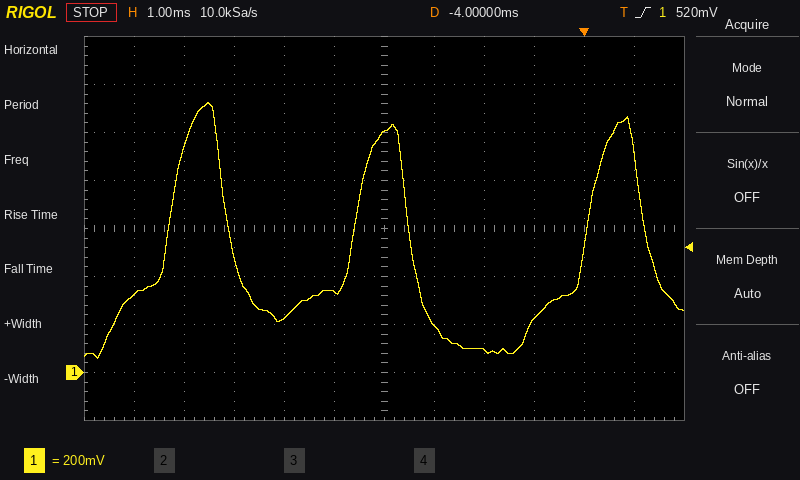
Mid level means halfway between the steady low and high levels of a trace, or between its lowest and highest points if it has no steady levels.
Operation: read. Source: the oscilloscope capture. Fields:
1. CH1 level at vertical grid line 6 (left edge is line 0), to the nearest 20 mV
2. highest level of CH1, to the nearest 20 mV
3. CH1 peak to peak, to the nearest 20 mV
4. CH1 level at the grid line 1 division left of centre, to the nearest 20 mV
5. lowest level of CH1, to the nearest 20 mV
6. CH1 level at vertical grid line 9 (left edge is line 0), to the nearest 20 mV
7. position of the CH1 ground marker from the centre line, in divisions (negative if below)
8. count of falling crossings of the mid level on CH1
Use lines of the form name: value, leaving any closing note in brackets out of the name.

CH1 level at vertical grid line 6 (left edge is line 0), to the nearest 20 mV: 1.00 V
highest level of CH1, to the nearest 20 mV: 1.12 V
CH1 peak to peak, to the nearest 20 mV: 1.06 V
CH1 level at the grid line 1 division left of centre, to the nearest 20 mV: 340 mV
lowest level of CH1, to the nearest 20 mV: 60 mV
CH1 level at vertical grid line 9 (left edge is line 0), to the nearest 20 mV: 220 mV
position of the CH1 ground marker from the centre line, in divisions: -3.0 div
count of falling crossings of the mid level on CH1: 3
